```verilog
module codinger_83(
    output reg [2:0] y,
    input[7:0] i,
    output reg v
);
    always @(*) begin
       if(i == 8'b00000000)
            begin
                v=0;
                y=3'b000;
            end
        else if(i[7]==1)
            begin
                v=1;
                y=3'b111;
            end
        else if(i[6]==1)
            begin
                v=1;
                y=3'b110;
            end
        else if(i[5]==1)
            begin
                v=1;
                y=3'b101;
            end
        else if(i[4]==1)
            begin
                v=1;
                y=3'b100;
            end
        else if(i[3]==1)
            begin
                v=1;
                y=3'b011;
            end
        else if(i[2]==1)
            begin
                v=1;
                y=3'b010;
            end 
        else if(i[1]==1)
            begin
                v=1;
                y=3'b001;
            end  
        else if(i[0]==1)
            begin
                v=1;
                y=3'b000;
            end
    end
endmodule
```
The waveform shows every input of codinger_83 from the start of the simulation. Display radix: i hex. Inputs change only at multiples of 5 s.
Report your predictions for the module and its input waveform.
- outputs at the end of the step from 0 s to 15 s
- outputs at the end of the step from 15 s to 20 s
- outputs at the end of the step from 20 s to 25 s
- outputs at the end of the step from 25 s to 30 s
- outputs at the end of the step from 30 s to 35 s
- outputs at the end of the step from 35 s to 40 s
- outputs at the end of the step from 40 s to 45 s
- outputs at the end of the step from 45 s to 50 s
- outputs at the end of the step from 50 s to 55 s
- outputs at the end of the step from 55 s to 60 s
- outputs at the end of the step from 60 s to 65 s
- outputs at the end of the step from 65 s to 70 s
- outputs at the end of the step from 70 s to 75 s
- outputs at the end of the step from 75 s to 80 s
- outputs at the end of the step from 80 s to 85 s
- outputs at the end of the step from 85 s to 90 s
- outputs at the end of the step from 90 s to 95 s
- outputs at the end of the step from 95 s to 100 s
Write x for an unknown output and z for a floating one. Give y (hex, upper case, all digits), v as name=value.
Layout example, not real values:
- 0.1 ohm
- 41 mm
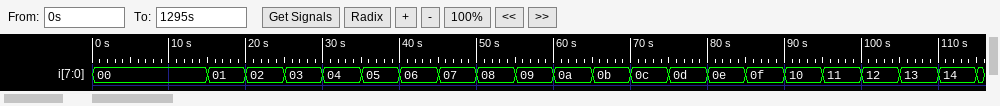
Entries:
- y=0, v=0
- y=0, v=1
- y=1, v=1
- y=1, v=1
- y=2, v=1
- y=2, v=1
- y=2, v=1
- y=2, v=1
- y=3, v=1
- y=3, v=1
- y=3, v=1
- y=3, v=1
- y=3, v=1
- y=3, v=1
- y=3, v=1
- y=3, v=1
- y=4, v=1
- y=4, v=1
